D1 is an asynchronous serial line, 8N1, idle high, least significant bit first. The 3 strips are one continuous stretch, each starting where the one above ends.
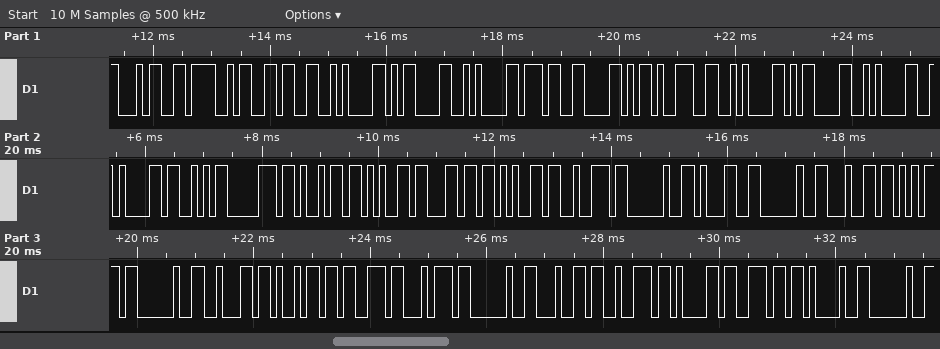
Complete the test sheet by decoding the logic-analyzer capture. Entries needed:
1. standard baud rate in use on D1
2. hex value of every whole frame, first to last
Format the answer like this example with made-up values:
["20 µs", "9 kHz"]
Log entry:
["9600 baud", "34 4F 36 0A 0D 0A 37 58 39 0A 0D 0A 0A 53 70 69 65 6C 65 72 20 31 20 64 75 20 62 69 73 74 20 64 72 61 6E 21 20"]
